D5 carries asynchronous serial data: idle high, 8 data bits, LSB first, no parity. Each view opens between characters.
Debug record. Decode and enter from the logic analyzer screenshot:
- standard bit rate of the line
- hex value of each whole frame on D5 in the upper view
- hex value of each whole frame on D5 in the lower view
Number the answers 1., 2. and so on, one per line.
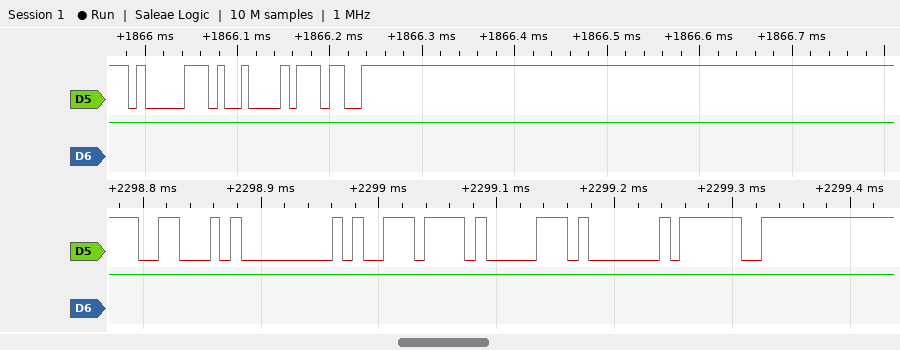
1. 115200 baud
2. C1, 09, 37
3. 46, 00, B9, C1, 01, 3F
